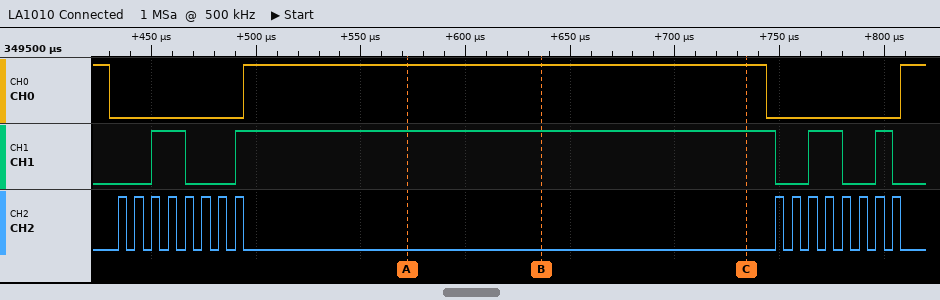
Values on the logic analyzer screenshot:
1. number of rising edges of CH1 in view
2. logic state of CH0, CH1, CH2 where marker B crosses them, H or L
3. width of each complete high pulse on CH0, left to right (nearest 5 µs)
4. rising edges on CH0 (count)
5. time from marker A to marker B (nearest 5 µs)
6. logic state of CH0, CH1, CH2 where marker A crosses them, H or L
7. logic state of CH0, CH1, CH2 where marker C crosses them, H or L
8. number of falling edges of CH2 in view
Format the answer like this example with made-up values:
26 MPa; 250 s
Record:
4; CH0=H, CH1=H, CH2=L; 250 µs; 2; 65 µs; CH0=H, CH1=H, CH2=L; CH0=H, CH1=H, CH2=L; 16
